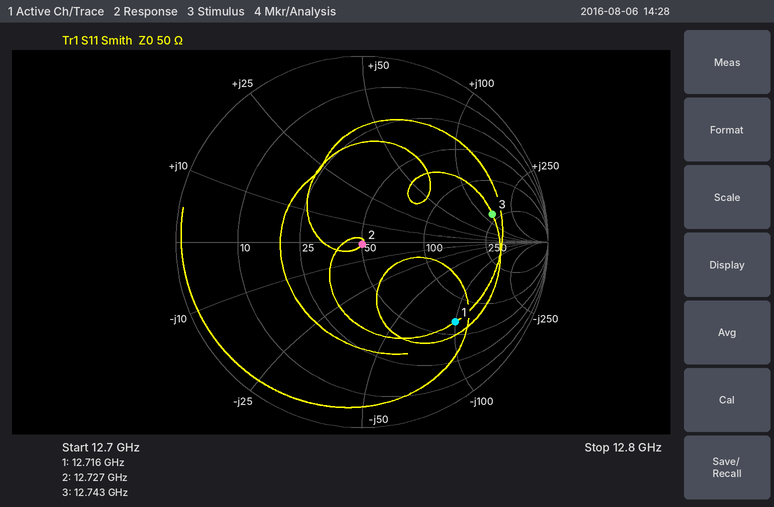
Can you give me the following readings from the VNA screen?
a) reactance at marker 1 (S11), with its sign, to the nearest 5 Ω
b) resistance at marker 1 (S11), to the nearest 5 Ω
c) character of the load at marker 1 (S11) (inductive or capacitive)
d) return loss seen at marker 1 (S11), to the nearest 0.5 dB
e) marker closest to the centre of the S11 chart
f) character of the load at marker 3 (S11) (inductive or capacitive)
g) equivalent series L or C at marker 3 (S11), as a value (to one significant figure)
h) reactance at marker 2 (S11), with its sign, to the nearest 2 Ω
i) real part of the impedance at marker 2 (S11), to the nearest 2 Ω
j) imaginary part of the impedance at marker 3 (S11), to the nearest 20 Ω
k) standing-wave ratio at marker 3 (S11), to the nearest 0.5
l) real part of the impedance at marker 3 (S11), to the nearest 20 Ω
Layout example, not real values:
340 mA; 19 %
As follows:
-100 Ω; 65 Ω; capacitive; 3.5 dB; marker 2; inductive; 2 nH; -2 Ω; 50 Ω; +140 Ω; 6.0; 220 Ω
